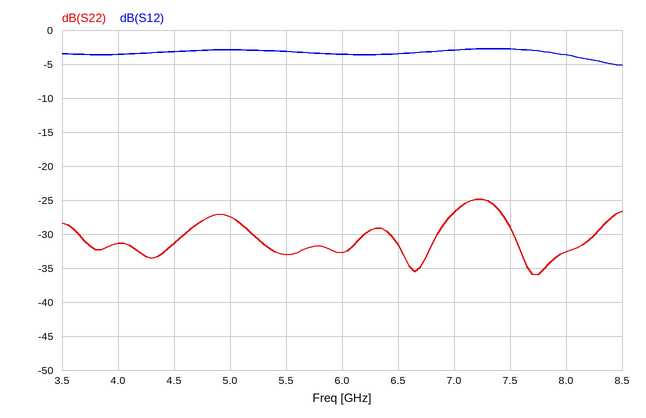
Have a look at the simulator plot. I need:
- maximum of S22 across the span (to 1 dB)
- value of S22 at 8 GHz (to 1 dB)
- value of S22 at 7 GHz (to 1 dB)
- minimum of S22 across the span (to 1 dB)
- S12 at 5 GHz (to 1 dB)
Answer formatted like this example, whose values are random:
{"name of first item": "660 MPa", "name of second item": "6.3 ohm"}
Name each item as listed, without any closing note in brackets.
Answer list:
{"maximum of S22 across the span": "-25 dB", "value of S22 at 8 GHz": "-33 dB", "value of S22 at 7 GHz": "-27 dB", "minimum of S22 across the span": "-36 dB", "S12 at 5 GHz": "-3 dB"}
